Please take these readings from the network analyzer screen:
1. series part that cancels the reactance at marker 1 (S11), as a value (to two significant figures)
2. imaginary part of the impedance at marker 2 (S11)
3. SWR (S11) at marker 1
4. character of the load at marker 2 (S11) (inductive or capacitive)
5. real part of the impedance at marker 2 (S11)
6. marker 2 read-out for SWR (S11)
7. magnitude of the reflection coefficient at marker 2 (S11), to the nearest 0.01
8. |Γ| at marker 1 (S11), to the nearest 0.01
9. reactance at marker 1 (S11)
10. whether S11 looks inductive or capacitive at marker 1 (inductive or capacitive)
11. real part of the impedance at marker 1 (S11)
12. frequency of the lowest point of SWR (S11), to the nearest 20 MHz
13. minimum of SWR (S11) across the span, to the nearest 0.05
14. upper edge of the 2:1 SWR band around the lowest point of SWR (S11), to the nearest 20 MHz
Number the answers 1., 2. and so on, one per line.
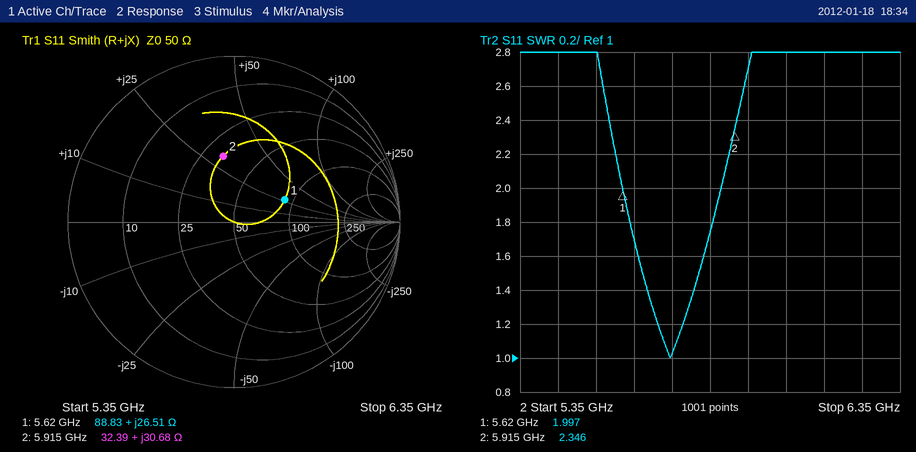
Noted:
1. 1.1 pF
2. +30.68 Ω
3. 1.997
4. inductive
5. 32.39 Ω
6. 2.346
7. 0.40
8. 0.33
9. +26.51 Ω
10. inductive
11. 88.83 Ω
12. 5.74 GHz
13. 1.00
14. 5.88 GHz
